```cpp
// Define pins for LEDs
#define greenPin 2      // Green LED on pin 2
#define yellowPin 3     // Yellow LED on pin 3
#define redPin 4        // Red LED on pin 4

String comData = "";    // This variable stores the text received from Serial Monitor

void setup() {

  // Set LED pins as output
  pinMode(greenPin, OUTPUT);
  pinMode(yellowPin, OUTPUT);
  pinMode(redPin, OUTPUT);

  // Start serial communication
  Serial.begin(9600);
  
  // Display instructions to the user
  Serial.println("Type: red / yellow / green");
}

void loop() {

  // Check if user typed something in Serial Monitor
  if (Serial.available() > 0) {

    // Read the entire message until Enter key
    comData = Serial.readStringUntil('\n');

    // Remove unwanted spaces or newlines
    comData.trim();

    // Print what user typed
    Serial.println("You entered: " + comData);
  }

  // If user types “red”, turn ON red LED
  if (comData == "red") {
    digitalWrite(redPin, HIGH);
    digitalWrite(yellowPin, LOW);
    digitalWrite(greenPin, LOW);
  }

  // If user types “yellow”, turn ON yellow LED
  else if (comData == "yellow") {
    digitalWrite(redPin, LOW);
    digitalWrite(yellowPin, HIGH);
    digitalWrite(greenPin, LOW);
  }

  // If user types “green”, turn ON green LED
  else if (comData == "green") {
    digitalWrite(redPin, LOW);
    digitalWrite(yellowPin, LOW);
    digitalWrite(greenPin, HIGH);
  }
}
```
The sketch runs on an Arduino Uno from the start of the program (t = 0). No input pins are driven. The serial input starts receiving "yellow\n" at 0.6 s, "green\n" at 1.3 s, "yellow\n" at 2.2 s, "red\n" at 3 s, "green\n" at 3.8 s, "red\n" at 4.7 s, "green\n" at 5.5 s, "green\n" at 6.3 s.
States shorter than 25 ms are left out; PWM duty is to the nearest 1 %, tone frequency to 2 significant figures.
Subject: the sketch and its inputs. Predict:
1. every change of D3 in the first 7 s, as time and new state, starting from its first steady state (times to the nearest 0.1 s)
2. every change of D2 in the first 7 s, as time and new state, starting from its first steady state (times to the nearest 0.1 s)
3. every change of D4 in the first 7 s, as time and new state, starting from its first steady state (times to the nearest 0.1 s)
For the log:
0 s low; 0.6 s high; 1.3 s low; 2.2 s high; 3 s low
0 s low; 1.3 s high; 2.2 s low; 3.8 s high; 4.7 s low; 5.5 s high
0 s low; 3 s high; 3.8 s low; 4.7 s high; 5.5 s low
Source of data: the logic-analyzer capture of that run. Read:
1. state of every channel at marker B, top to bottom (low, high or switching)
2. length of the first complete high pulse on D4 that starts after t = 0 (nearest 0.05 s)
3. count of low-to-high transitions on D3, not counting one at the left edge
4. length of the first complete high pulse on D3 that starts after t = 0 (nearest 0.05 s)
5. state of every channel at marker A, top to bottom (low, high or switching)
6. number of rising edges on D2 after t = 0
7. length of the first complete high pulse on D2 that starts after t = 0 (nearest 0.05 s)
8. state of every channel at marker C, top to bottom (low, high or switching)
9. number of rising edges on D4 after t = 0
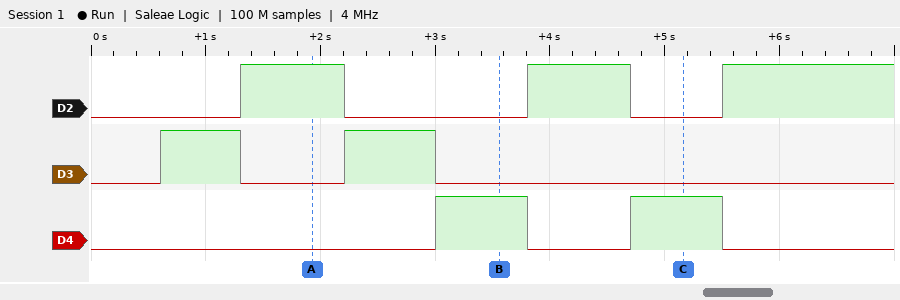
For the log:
D2 low, D3 low, D4 high
0.80 s
2
0.70 s
D2 high, D3 low, D4 low
3
0.90 s
D2 low, D3 low, D4 high
2
